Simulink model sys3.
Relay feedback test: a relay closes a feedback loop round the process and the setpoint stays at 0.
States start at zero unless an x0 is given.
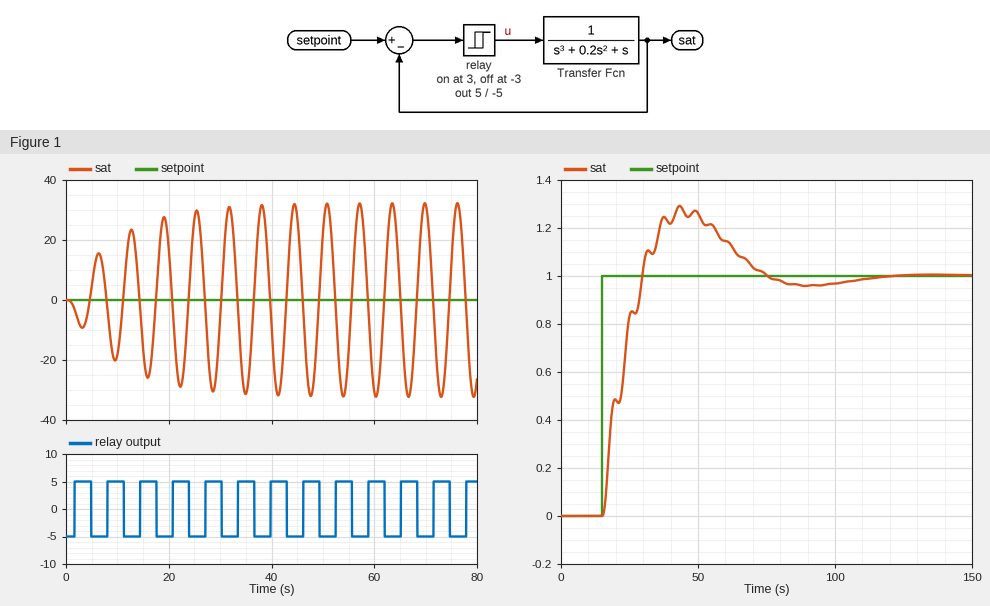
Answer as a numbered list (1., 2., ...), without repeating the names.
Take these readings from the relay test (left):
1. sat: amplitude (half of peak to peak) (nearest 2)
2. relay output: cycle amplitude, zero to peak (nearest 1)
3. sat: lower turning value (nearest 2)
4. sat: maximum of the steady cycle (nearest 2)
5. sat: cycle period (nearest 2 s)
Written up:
1. 32
2. 5
3. -32
4. 32
5. 6 s
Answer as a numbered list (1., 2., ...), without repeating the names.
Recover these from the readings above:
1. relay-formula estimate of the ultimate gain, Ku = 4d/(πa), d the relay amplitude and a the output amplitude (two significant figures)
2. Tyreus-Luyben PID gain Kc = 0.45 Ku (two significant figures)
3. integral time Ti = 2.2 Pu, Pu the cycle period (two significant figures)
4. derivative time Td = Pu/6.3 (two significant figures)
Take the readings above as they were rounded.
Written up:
1. 0.20
2. 0.090
3. 13 s
4. 0.95 s
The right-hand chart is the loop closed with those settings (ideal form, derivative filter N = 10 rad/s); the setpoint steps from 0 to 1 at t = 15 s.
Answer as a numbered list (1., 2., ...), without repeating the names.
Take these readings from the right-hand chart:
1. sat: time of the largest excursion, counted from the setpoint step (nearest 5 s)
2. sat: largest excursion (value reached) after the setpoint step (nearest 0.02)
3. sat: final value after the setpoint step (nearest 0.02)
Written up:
1. 30 s
2. 1.30
3. 1.00
